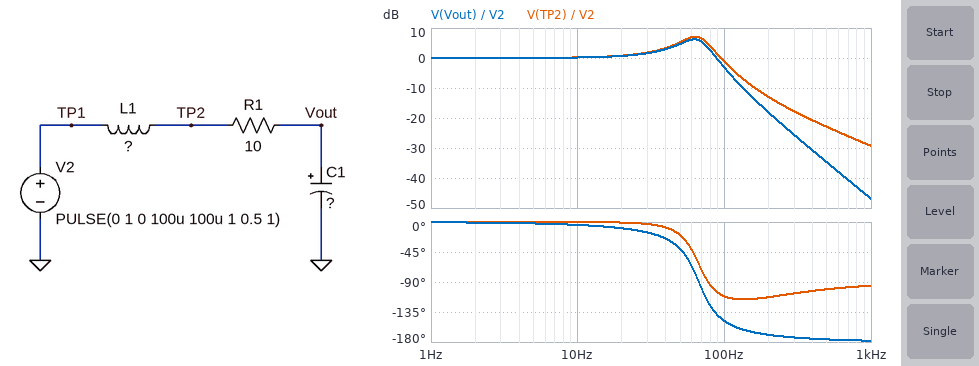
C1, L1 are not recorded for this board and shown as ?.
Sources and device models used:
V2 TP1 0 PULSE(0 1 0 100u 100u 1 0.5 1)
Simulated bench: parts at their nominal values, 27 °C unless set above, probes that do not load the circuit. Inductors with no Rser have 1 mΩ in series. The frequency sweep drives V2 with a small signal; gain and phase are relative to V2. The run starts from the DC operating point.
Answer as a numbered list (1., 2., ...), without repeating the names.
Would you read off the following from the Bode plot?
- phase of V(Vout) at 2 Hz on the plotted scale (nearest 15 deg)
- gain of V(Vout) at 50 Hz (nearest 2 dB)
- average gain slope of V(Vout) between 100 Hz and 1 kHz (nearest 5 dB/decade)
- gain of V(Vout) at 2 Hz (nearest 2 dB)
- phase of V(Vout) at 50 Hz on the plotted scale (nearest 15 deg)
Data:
1. 0 deg
2. 4 dB
3. -45 dB/decade
4. 0 dB
5. -45 deg
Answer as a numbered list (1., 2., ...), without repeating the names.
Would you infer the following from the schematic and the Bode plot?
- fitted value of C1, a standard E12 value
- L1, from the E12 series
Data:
1. 120 µF
2. 47 mH
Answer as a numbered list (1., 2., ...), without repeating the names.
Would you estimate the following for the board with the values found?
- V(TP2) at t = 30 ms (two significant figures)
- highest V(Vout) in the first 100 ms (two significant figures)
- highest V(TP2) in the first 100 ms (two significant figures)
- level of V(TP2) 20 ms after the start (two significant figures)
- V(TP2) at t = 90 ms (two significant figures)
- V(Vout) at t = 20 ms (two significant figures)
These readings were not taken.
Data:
1. 960 mV
2. 1.4 V
3. 1.5 V
4. 1.1 V
5. 1.0 V
6. 1.0 V
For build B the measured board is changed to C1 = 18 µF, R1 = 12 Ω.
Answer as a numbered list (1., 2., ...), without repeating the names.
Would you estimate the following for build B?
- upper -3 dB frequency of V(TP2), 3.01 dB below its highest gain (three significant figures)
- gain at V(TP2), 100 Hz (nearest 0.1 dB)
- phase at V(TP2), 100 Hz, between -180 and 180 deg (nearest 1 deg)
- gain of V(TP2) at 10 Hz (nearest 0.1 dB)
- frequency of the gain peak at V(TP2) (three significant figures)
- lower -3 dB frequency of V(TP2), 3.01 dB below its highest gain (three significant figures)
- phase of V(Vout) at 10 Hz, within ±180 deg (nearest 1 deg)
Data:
1. 190 Hz
2. 3.4 dB
3. -4 deg
4. 0 dB
5. 171 Hz
6. 149 Hz
7. -1 deg
